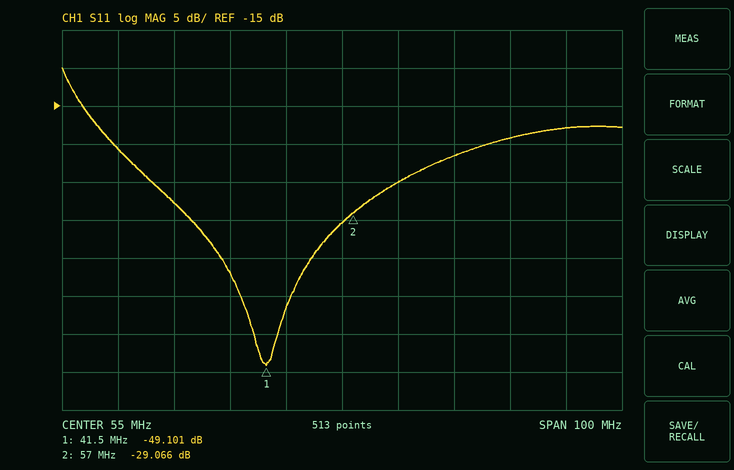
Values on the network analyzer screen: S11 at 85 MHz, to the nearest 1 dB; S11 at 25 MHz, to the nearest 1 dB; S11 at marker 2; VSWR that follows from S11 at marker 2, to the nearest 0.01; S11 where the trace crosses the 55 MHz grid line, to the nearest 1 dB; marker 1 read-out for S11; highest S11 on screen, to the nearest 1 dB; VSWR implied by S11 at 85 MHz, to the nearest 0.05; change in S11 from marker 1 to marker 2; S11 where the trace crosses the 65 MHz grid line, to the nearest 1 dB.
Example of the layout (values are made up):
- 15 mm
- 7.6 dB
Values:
- -19 dB
- -28 dB
- -29.066 dB
- 1.07
- -30 dB
- -49.101 dB
- -10 dB
- 1.25
- 20.035 dB
- -25 dB
